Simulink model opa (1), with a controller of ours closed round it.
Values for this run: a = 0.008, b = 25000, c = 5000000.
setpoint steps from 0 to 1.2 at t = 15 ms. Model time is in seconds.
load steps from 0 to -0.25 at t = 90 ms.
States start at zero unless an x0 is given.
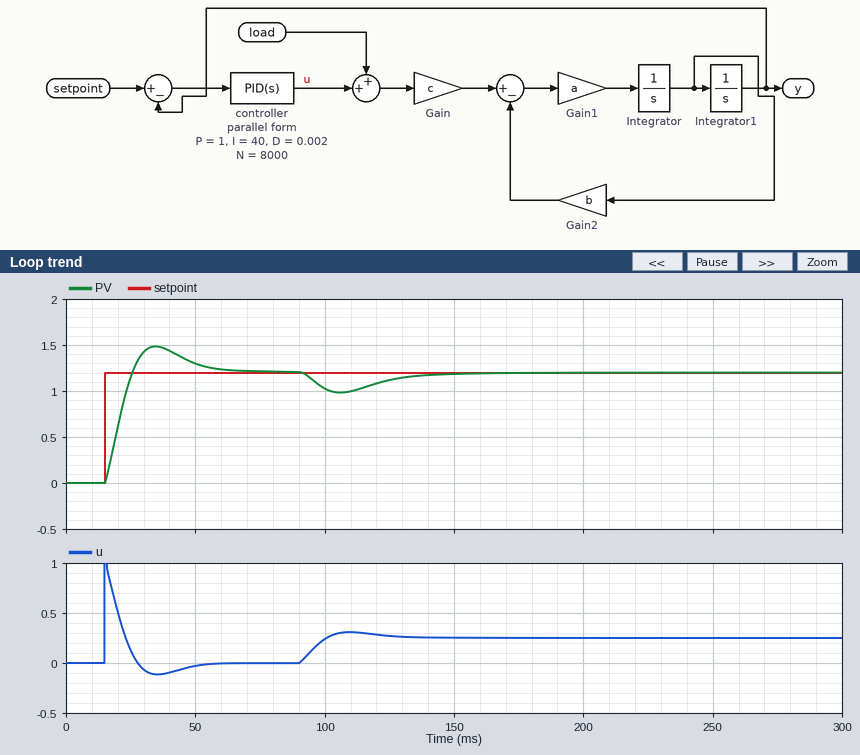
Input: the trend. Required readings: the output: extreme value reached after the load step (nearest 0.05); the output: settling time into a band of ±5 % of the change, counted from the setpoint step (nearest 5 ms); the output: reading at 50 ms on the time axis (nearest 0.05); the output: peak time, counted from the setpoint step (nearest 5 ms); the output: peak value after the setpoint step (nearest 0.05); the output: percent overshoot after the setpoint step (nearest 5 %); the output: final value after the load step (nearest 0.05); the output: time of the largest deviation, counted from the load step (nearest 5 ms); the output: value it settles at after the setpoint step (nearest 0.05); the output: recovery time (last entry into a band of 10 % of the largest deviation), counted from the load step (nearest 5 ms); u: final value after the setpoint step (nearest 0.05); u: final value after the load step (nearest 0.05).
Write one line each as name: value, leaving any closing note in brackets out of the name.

the output: extreme value reached after the load step: 1.00
the output: settling time into a band of ±5 % of the change, counted from the setpoint step: 40 ms
the output: reading at 50 ms on the time axis: 1.30
the output: peak time, counted from the setpoint step: 20 ms
the output: peak value after the setpoint step: 1.50
the output: percent overshoot after the setpoint step: 25 %
the output: final value after the load step: 1.20
the output: time of the largest deviation, counted from the load step: 15 ms
the output: value it settles at after the setpoint step: 1.20
the output: recovery time (last entry into a band of 10 % of the largest deviation), counted from the load step: 55 ms
u: final value after the setpoint step: 0.00
u: final value after the load step: 0.25
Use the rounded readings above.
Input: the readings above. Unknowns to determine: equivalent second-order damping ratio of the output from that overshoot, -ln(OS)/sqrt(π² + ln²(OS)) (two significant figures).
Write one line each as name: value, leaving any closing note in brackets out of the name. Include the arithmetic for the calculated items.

equivalent second-order damping ratio of the output from that overshoot, -ln(OS)/sqrt(π² + ln²(OS)): ln(0.25) = -1.386; 1.386 / sqrt(9.870 + 1.922) = 0.40
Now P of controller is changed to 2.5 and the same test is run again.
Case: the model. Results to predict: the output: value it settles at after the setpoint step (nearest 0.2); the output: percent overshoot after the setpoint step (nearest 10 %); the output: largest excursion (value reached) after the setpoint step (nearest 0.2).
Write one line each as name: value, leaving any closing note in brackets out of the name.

the output: value it settles at after the setpoint step: 1.2
the output: percent overshoot after the setpoint step: 30 %
the output: largest excursion (value reached) after the setpoint step: 1.6
